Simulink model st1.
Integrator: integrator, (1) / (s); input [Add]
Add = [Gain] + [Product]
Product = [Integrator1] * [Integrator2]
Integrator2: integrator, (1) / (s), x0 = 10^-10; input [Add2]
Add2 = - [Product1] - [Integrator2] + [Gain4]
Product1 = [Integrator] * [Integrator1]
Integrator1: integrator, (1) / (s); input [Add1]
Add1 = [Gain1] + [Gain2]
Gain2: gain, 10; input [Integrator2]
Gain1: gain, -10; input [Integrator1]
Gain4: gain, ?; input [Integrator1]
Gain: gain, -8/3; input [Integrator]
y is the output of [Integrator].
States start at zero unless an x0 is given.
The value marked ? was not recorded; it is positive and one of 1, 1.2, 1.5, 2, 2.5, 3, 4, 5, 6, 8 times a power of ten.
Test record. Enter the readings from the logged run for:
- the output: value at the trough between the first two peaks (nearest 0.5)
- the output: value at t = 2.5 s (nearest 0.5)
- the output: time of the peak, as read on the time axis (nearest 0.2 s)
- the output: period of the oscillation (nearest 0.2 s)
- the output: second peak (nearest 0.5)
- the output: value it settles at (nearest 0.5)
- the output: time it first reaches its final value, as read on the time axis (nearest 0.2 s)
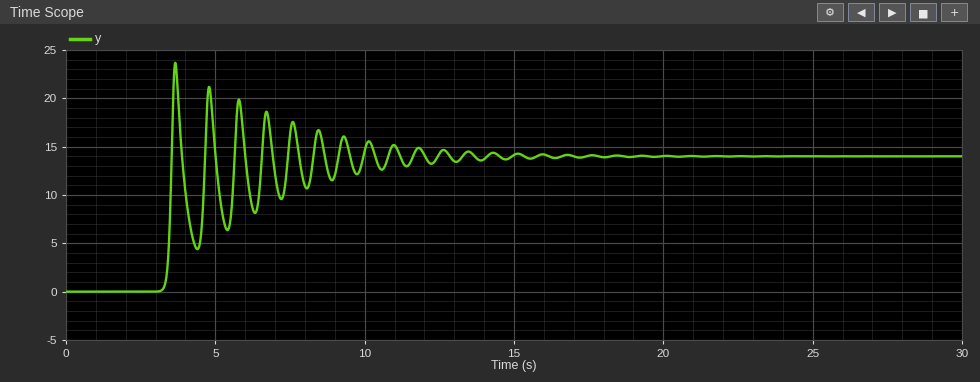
4.5
0.0
3.6 s
1.2 s
21.0
14.0
3.6 s
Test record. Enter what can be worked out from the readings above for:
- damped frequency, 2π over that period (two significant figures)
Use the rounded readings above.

5.2 rad/s
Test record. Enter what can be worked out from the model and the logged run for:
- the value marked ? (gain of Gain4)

15
